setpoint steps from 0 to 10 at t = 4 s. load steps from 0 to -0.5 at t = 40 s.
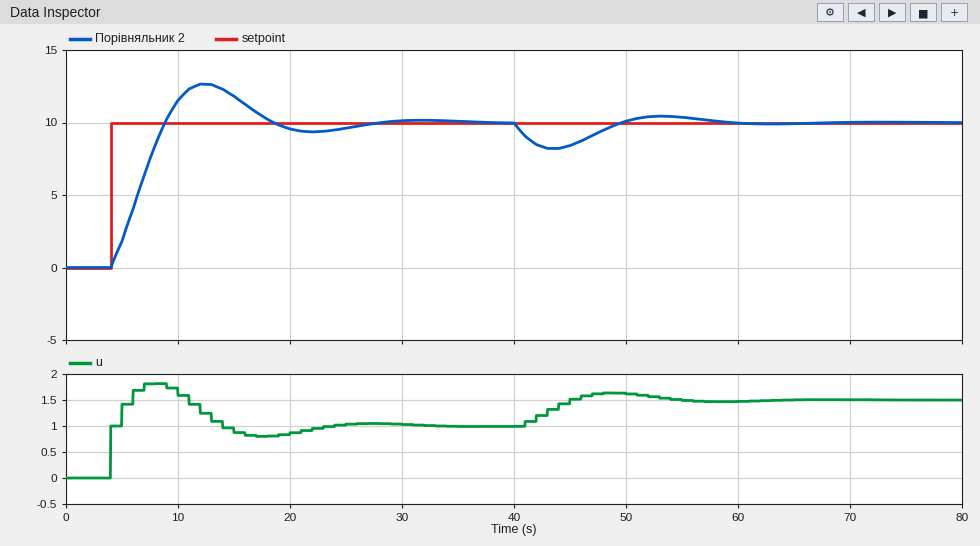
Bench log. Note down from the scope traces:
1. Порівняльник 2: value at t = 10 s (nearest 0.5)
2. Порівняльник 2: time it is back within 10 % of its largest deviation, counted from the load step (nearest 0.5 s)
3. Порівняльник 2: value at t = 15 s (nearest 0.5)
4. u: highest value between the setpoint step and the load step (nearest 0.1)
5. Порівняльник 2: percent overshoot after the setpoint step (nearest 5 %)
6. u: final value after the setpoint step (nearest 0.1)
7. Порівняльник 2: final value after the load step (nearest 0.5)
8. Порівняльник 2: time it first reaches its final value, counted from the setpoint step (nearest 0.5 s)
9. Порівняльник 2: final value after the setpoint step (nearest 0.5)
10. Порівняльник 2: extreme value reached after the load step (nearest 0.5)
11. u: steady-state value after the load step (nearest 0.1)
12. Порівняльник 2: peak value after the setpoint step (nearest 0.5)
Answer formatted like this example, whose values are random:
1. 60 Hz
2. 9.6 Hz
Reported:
1. 11.5
2. 17.0 s
3. 12.0
4. 1.8
5. 25 %
6. 1.0
7. 10.0
8. 5.0 s
9. 10.0
10. 8.0
11. 1.5
12. 12.5
